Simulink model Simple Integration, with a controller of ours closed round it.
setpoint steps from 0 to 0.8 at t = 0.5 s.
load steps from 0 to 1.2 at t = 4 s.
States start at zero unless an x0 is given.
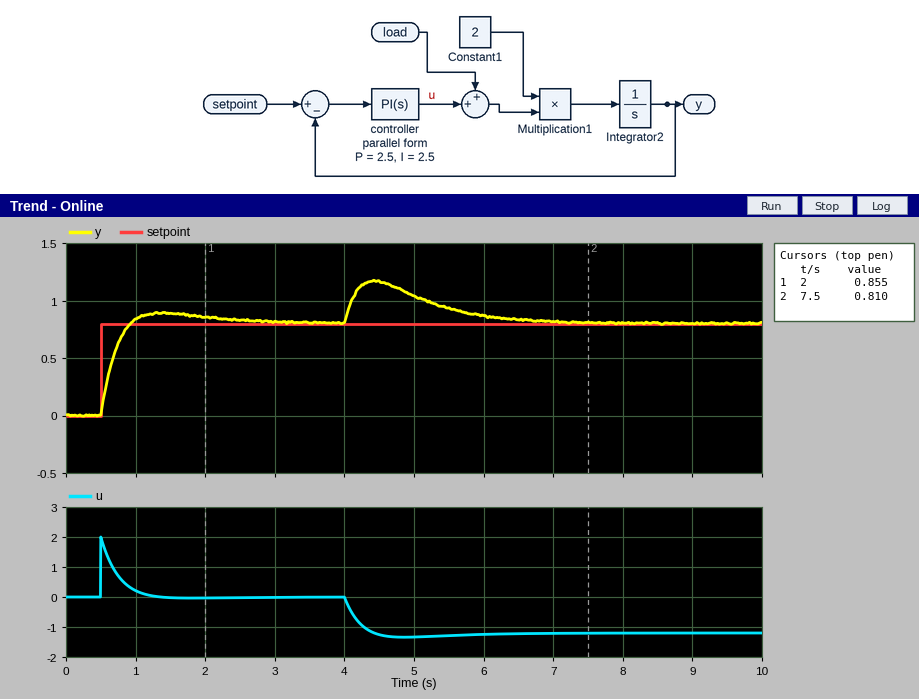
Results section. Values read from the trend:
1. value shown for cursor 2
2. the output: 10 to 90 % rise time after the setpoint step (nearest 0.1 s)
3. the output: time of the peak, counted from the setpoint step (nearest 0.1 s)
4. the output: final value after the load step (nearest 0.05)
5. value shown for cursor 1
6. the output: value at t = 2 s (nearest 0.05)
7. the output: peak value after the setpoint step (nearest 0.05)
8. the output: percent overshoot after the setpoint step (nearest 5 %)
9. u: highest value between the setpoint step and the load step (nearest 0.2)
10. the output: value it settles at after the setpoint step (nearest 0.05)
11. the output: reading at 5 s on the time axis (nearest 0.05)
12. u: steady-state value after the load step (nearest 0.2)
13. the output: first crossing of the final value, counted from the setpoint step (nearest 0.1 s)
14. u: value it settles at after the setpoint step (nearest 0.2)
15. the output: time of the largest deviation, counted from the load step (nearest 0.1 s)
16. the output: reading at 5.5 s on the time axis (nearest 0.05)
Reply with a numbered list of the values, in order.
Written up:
1. 0.810
2. 0.3 s
3. 0.9 s
4. 0.80
5. 0.855
6. 0.85
7. 0.90
8. 10 %
9. 2.0
10. 0.80
11. 1.05
12. -1.2
13. 0.4 s
14. 0.0
15. 0.4 s
16. 0.95
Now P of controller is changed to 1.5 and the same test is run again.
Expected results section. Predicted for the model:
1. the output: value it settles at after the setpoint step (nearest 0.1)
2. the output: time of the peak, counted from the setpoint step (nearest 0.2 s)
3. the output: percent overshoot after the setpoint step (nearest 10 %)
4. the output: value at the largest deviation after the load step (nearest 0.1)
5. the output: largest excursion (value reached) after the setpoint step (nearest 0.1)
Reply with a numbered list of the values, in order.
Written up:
1. 0.8
2. 1.0 s
3. 20 %
4. 1.3
5. 1.0
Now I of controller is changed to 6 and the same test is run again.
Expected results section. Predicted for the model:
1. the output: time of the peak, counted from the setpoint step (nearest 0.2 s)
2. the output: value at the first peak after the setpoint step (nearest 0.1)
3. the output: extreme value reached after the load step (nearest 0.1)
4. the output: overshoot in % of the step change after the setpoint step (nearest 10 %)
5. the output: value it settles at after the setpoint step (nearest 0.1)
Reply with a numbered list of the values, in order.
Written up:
1. 0.6 s
2. 1.0
3. 1.1
4. 20 %
5. 0.8
